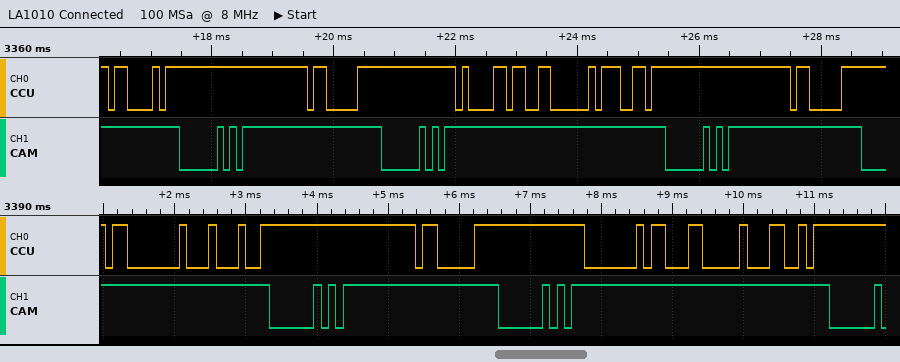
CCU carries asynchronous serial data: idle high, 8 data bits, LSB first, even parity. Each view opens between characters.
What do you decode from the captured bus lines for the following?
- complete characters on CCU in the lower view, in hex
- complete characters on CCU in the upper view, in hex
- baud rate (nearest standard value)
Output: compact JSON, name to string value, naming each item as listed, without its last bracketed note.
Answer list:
{"complete characters on CCU in the lower view, in hex": "03, 44, 83, 40, 0C, 4C", "complete characters on CCU in the upper view, in hex": "43, 83, 61, 06, 67, 83", "baud rate": "9600 baud"}
